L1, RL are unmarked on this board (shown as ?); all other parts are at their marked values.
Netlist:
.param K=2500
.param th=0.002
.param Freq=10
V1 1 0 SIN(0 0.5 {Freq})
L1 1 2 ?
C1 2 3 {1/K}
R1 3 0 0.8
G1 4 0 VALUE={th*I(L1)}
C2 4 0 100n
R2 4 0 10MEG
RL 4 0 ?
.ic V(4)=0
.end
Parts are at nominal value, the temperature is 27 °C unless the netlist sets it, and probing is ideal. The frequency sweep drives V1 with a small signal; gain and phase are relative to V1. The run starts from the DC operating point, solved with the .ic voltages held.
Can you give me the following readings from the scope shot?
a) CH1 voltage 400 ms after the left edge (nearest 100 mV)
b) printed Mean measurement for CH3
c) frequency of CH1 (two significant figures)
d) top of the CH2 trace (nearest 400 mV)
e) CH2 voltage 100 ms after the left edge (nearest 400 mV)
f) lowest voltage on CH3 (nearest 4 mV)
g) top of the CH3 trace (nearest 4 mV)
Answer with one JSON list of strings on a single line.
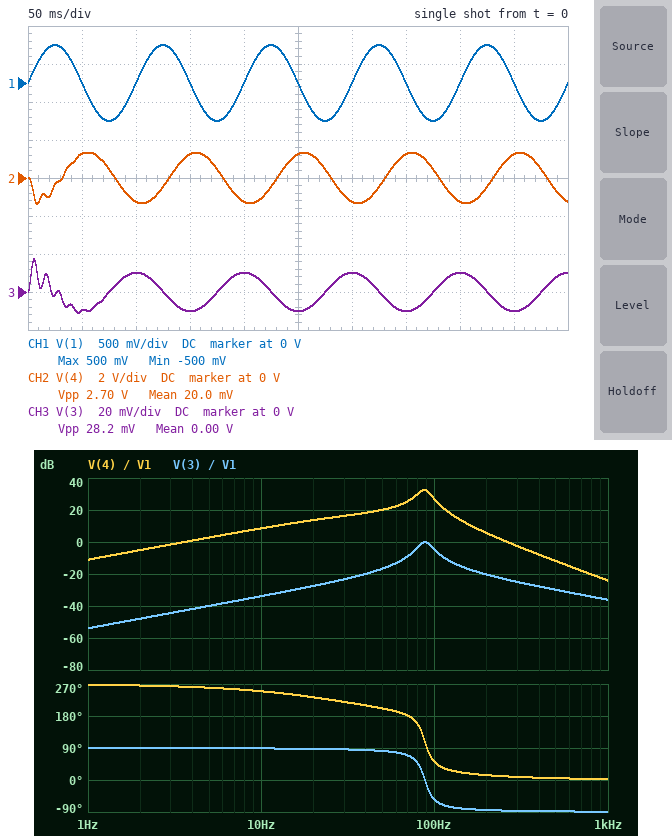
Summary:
["0 V", "0.00 V", "10 Hz", "1.2 V", "-1.2 V", "-12 mV", "16 mV"]
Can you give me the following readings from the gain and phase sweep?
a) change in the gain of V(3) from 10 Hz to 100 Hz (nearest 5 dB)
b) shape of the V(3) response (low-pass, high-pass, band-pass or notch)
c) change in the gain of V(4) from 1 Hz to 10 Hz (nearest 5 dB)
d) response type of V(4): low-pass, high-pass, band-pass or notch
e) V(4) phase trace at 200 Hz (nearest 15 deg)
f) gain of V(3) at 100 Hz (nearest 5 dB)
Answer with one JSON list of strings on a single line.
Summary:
["30 dB", "band-pass", "20 dB", "band-pass", "15 deg", "-5 dB"]
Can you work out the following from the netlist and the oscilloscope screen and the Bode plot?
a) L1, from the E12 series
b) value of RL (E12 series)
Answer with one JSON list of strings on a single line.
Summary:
["8.2 mH", "56 kΩ"]
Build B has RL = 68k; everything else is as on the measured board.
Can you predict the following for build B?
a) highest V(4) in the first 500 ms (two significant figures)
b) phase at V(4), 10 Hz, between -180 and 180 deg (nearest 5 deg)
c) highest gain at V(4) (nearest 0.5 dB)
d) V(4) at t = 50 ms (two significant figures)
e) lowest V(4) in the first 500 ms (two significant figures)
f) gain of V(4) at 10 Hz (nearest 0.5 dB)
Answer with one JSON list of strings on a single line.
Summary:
["1.6 V", "-115 deg", "33.0 dB", "1.5 V", "-1.6 V", "10.0 dB"]
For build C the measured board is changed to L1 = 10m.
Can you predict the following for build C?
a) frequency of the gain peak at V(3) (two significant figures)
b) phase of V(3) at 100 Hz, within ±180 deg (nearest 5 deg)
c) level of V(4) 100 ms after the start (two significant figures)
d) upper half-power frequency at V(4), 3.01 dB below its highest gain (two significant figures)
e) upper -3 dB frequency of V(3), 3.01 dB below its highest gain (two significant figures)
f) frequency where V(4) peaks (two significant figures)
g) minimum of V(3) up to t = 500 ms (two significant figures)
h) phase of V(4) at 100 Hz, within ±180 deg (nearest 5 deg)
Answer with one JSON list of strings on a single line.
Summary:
["80 Hz", "-70 deg", "-1.3 V", "85 Hz", "86 Hz", "79 Hz", "-12 mV", "35 deg"]
